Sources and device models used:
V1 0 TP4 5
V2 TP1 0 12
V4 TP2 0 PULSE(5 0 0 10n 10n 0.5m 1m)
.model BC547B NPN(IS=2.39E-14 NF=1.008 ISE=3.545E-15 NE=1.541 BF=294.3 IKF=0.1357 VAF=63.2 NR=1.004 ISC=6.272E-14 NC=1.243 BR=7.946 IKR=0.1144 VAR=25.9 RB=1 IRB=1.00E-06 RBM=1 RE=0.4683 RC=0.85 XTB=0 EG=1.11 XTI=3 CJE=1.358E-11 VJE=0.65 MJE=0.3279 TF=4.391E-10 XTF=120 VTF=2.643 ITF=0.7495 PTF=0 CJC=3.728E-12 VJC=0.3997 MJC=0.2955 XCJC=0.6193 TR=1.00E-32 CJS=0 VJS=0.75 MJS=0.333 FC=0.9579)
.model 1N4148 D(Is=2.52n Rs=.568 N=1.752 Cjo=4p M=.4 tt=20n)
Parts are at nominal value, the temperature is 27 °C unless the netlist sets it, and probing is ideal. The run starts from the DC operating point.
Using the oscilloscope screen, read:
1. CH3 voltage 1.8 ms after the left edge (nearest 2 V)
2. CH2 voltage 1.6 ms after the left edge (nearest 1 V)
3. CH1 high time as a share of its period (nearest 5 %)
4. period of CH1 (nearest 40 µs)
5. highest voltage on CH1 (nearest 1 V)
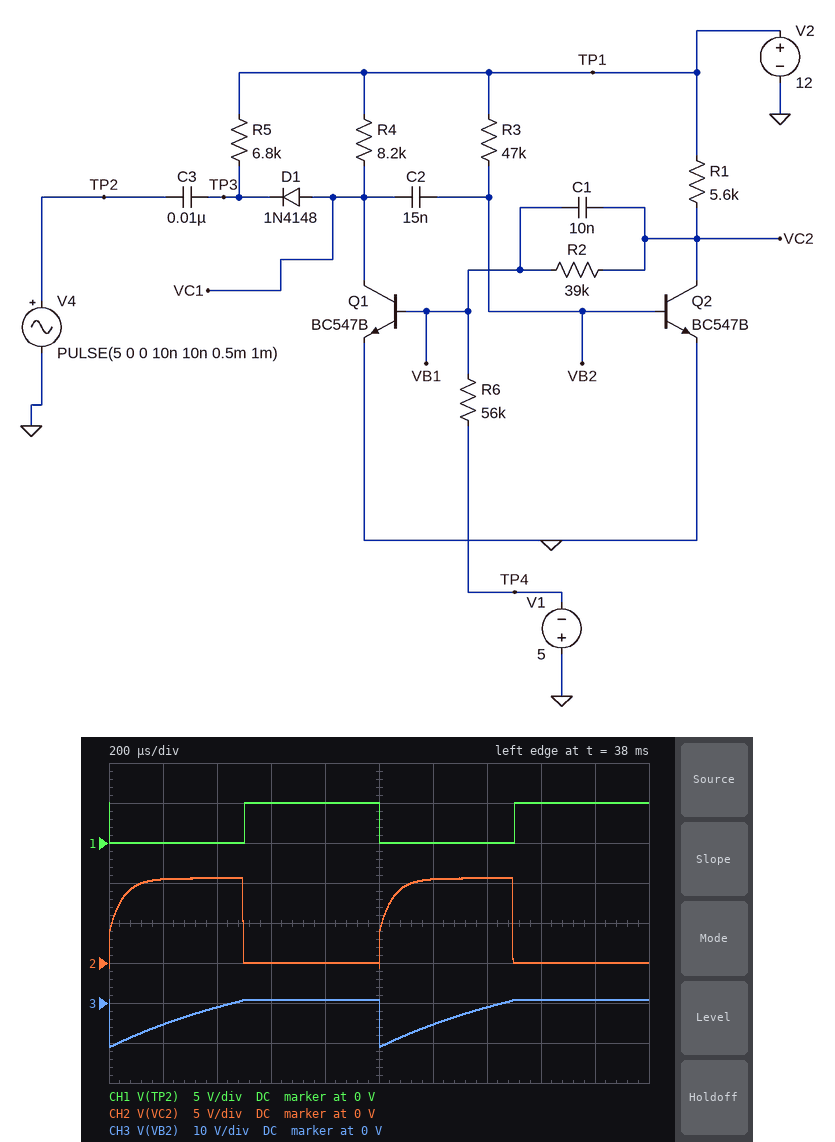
0 V
0 V
50 %
1.00 ms
5 V
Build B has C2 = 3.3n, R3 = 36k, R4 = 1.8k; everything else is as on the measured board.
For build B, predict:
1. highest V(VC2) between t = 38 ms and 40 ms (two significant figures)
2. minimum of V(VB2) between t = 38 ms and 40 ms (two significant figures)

9.2 V
-11 V
